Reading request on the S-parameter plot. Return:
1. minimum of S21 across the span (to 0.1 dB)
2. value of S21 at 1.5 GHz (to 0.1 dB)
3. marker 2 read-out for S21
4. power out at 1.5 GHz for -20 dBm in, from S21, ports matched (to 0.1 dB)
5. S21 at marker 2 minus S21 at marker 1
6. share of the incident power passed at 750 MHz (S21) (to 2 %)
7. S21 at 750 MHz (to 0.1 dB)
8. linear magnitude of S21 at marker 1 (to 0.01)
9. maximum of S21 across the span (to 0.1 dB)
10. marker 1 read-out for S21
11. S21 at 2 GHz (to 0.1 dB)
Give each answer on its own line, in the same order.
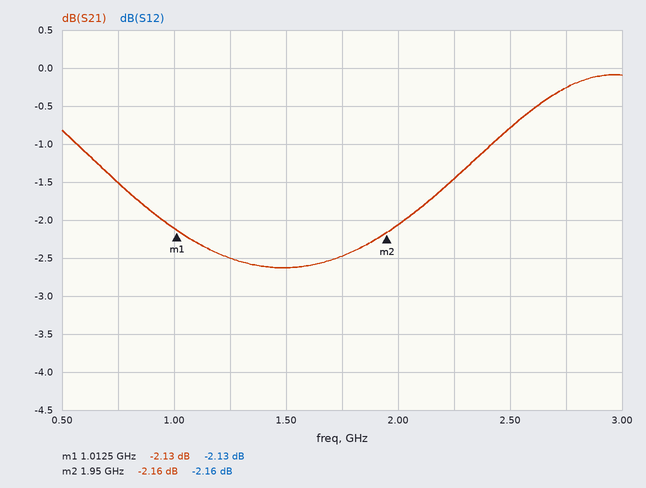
-2.6 dB
-2.6 dB
-2.16 dB
-22.6 dBm
-0.03 dB
70 %
-1.5 dB
0.78
-0.1 dB
-2.13 dB
-2.1 dB
